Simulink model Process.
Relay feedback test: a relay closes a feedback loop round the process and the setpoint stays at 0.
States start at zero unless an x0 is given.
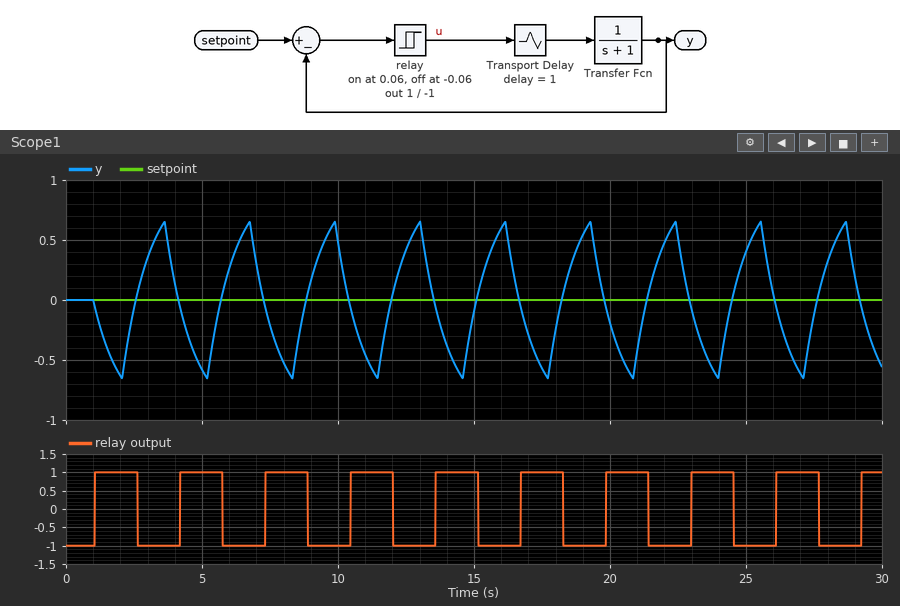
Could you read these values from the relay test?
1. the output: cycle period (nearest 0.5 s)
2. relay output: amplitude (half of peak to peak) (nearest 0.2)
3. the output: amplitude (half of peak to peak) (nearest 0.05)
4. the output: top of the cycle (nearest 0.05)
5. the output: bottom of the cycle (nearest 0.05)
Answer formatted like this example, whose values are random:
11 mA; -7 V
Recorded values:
3.0 s; 1.0; 0.65; 0.65; -0.65
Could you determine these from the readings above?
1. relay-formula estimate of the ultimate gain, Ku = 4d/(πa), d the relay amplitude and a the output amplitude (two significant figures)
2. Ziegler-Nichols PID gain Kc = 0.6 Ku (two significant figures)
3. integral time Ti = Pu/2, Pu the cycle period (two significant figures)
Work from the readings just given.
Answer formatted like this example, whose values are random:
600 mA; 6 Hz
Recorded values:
2.0; 1.2; 1.5 s
